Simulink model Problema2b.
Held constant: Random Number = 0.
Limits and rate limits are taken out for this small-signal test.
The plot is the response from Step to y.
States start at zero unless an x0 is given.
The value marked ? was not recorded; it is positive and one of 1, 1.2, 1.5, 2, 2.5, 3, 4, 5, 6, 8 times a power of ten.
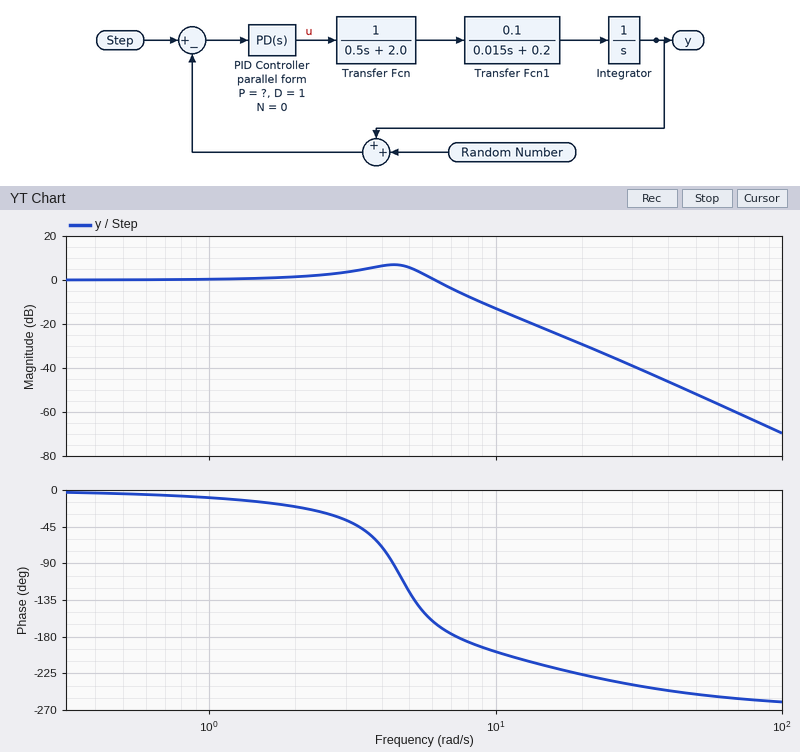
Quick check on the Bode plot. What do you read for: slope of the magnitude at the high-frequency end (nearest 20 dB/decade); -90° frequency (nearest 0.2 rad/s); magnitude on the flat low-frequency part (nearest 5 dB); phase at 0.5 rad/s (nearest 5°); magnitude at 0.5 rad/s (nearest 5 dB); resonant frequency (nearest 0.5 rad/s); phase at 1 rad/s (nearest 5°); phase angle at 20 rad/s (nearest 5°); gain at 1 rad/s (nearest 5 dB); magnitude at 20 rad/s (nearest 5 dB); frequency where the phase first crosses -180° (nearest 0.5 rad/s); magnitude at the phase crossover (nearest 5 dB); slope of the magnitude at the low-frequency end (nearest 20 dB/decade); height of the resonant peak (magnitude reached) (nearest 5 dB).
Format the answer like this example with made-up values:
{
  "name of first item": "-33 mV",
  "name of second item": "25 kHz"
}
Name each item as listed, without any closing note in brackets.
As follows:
{
  "slope of the magnitude at the high-frequency end": "-60 dB/decade",
  "-90° frequency": "4.4 rad/s",
  "magnitude on the flat low-frequency part": "0 dB",
  "phase at 0.5 rad/s": "-5°",
  "magnitude at 0.5 rad/s": "0 dB",
  "resonant frequency": "4.5 rad/s",
  "phase at 1 rad/s": "-10°",
  "phase angle at 20 rad/s": "-225°",
  "gain at 1 rad/s": "0 dB",
  "magnitude at 20 rad/s": "-30 dB",
  "frequency where the phase first crosses -180°": "7.5 rad/s",
  "magnitude at the phase crossover": "-5 dB",
  "slope of the magnitude at the low-frequency end": "0 dB/decade",
  "height of the resonant peak (magnitude reached)": "5 dB"
}
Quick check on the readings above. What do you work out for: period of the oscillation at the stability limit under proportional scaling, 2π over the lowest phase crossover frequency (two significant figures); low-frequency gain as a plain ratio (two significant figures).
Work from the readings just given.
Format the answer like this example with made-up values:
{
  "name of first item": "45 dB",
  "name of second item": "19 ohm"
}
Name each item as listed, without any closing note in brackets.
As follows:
{
  "period of the oscillation at the stability limit under proportional scaling, 2π over the lowest phase crossover frequency": "0.84 s",
  "low-frequency gain as a plain ratio": "1.0"
}
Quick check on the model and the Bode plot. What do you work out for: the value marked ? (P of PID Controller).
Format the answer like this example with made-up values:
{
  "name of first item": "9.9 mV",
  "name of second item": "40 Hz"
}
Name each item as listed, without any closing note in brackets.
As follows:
{
  "the value marked ?": "25"
}
